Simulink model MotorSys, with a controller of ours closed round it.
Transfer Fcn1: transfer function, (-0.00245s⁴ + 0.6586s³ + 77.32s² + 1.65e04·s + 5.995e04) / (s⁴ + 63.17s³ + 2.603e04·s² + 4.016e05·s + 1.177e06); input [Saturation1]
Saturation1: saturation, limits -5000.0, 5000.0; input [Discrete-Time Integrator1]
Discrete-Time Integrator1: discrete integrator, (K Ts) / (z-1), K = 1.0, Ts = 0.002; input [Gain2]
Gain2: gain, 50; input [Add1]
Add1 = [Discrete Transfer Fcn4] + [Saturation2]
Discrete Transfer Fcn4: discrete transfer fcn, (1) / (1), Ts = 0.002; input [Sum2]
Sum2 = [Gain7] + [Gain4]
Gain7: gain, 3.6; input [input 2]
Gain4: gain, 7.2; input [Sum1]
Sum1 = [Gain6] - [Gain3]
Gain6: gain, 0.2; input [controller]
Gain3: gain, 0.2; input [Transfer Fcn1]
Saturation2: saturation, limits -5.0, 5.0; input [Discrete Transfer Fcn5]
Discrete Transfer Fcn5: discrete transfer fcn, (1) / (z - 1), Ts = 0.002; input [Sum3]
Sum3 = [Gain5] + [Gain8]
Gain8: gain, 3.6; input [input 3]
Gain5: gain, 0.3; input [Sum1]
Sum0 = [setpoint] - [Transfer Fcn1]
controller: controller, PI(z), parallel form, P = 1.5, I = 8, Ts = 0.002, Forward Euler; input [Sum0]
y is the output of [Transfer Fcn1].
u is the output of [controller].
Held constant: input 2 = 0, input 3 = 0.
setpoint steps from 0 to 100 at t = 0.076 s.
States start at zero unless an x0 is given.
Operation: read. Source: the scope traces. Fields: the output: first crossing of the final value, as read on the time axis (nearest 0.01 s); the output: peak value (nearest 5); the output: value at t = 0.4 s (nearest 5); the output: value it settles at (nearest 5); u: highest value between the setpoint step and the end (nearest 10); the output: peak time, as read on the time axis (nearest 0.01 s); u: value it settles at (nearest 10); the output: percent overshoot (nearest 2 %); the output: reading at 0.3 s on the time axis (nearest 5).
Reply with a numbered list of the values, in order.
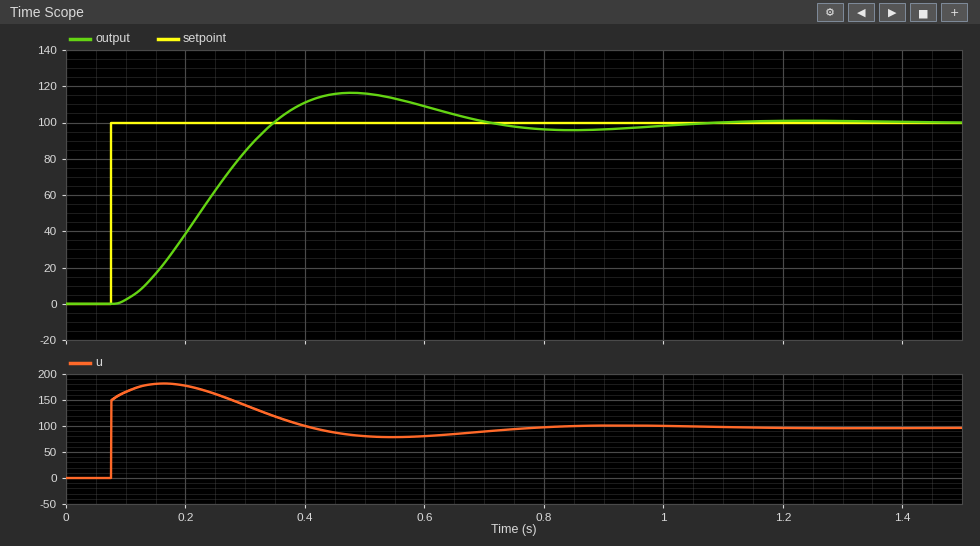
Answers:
1. 0.35 s
2. 115
3. 110
4. 100
5. 180
6. 0.48 s
7. 100
8. 16 %
9. 85
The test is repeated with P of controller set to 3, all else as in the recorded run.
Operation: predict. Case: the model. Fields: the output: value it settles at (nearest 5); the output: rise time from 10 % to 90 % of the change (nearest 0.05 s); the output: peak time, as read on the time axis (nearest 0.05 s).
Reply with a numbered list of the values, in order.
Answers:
1. 100
2. 0.15 s
3. 0.35 s
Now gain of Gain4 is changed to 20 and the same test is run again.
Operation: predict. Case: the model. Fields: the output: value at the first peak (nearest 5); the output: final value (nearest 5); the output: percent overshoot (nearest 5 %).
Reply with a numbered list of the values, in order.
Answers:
1. 110
2. 100
3. 10 %
